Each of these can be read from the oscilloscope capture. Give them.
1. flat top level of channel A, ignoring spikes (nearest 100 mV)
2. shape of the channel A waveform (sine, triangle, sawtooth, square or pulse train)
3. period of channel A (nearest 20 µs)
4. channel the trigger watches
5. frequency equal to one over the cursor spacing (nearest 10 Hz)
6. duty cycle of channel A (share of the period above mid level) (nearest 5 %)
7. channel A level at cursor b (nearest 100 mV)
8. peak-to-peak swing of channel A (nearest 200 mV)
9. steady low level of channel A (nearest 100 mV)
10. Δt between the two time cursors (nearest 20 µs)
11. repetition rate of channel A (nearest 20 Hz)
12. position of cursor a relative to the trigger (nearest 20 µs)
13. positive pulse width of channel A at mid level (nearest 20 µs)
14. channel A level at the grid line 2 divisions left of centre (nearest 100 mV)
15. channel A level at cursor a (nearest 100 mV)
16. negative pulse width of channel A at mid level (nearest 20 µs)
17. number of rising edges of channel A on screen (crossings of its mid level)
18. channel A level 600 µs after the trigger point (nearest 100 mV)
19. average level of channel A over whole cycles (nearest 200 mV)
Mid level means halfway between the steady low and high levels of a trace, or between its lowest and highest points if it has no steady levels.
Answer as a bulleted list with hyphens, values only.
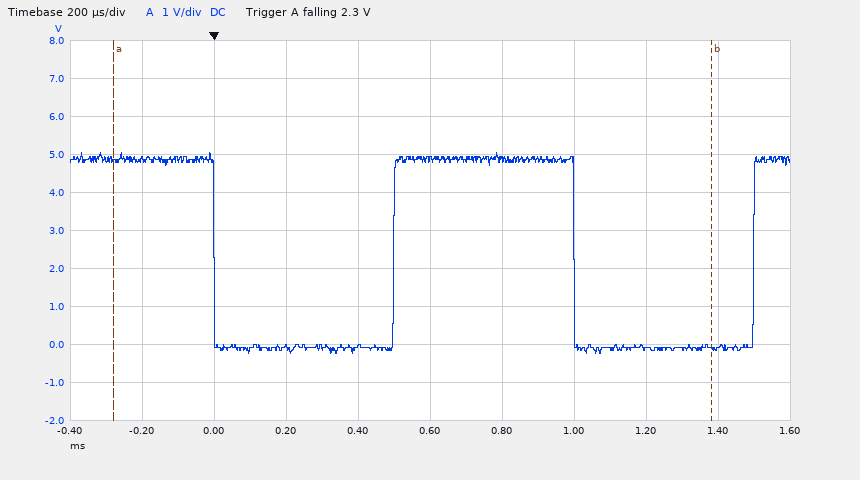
- 4.9 V
- square
- 1.00 ms
- channel A
- 600 Hz
- 50 %
- -100 mV
- 5.2 V
- -100 mV
- 1.66 ms
- 1.00 kHz
- -280 µs
- 500 µs
- -100 mV
- 4.9 V
- 500 µs
- 2
- 4.9 V
- 2.4 V
